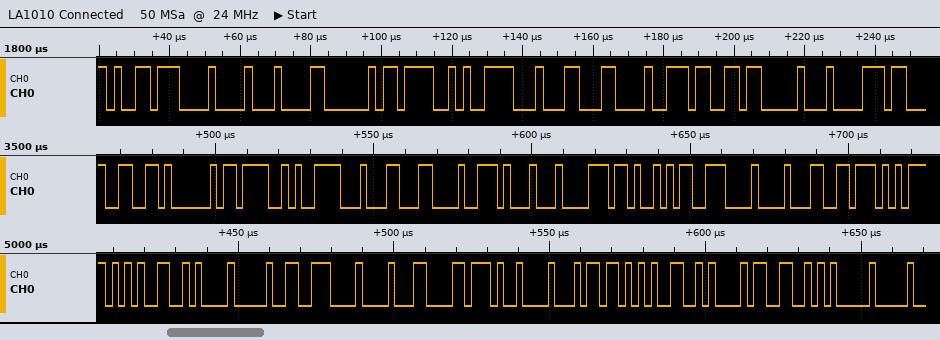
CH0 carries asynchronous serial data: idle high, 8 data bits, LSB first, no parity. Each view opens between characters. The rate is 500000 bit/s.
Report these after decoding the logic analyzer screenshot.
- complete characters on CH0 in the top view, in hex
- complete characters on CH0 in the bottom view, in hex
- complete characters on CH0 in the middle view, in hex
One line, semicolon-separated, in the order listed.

D9, 08, 84, A0, 4F, 1E, 8C, C8, B3, 10, B8; 95, 0A, 90, 0E, 88, D8, 09, B4, 95, 0A, 33, 05; 66, A0, 4F, 1E, 8C, C8, 11, B8, A9, 0E, 88, 76
